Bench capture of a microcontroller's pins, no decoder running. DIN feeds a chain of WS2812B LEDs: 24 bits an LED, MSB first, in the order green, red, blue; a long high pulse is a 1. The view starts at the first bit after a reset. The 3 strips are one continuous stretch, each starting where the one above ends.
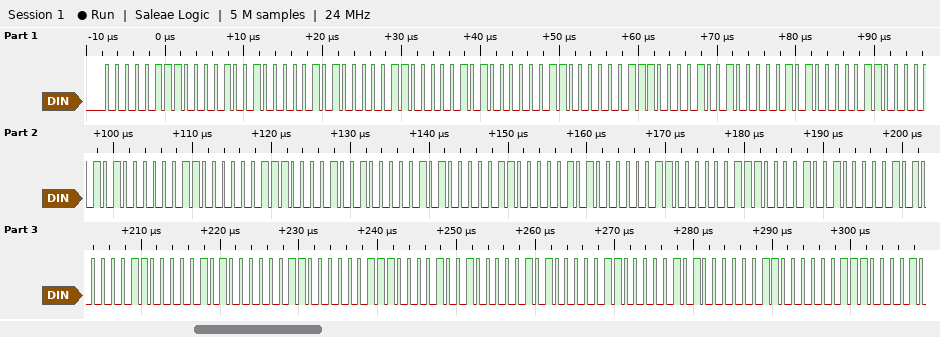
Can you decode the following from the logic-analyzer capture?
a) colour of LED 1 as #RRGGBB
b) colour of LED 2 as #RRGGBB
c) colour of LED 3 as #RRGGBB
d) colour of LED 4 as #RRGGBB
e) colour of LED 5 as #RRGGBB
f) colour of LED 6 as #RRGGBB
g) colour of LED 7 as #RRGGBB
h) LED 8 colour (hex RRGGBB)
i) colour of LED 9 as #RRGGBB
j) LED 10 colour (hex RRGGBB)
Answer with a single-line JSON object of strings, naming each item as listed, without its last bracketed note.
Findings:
{"colour of LED 1 as #RRGGBB": "#090705", "colour of LED 2 as #RRGGBB": "#0A0606", "colour of LED 3 as #RRGGBB": "#090705", "colour of LED 4 as #RRGGBB": "#0A0606", "colour of LED 5 as #RRGGBB": "#090705", "colour of LED 6 as #RRGGBB": "#0A0606", "colour of LED 7 as #RRGGBB": "#090705", "LED 8 colour": "#0A0606", "colour of LED 9 as #RRGGBB": "#090705", "LED 10 colour": "#0A0606"}
